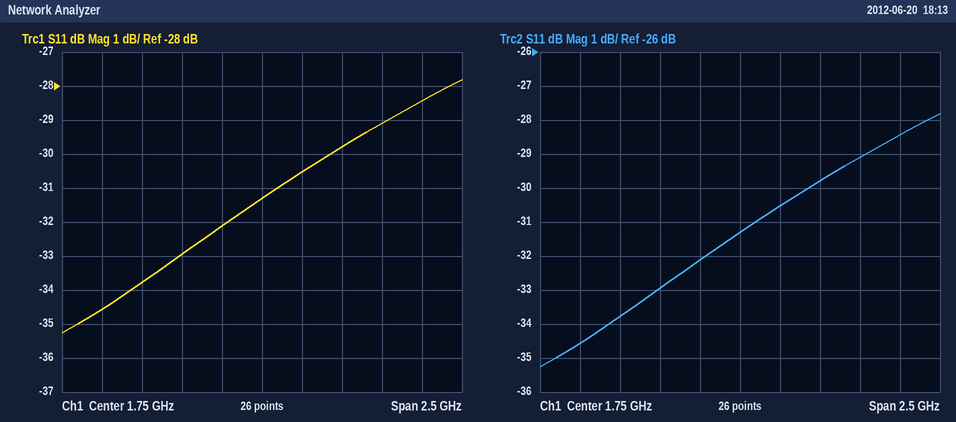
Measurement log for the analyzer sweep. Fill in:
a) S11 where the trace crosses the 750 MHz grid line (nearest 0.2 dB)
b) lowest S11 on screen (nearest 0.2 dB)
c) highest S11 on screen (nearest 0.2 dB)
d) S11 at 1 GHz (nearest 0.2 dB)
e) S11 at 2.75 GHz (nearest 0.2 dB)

-34.6 dB
-35.2 dB
-27.8 dB
-33.8 dB
-28.4 dB
